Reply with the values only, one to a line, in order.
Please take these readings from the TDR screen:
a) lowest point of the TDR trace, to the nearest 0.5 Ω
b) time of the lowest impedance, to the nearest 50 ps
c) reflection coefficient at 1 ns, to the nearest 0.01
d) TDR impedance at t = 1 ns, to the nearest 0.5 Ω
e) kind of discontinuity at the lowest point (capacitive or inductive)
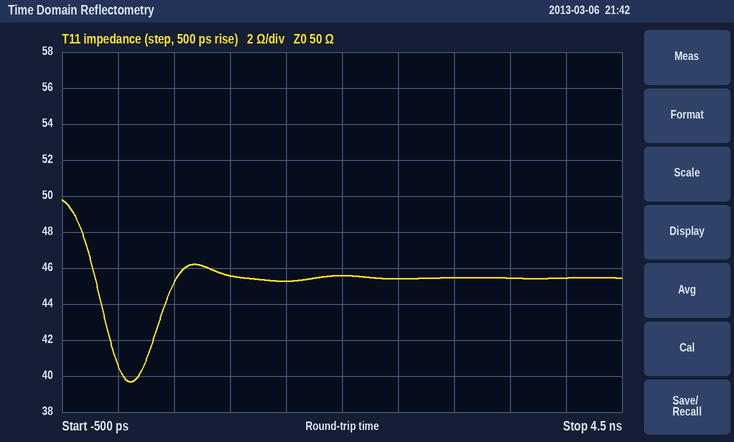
39.5 Ω
100 ps
-0.05
45.5 Ω
capacitive
